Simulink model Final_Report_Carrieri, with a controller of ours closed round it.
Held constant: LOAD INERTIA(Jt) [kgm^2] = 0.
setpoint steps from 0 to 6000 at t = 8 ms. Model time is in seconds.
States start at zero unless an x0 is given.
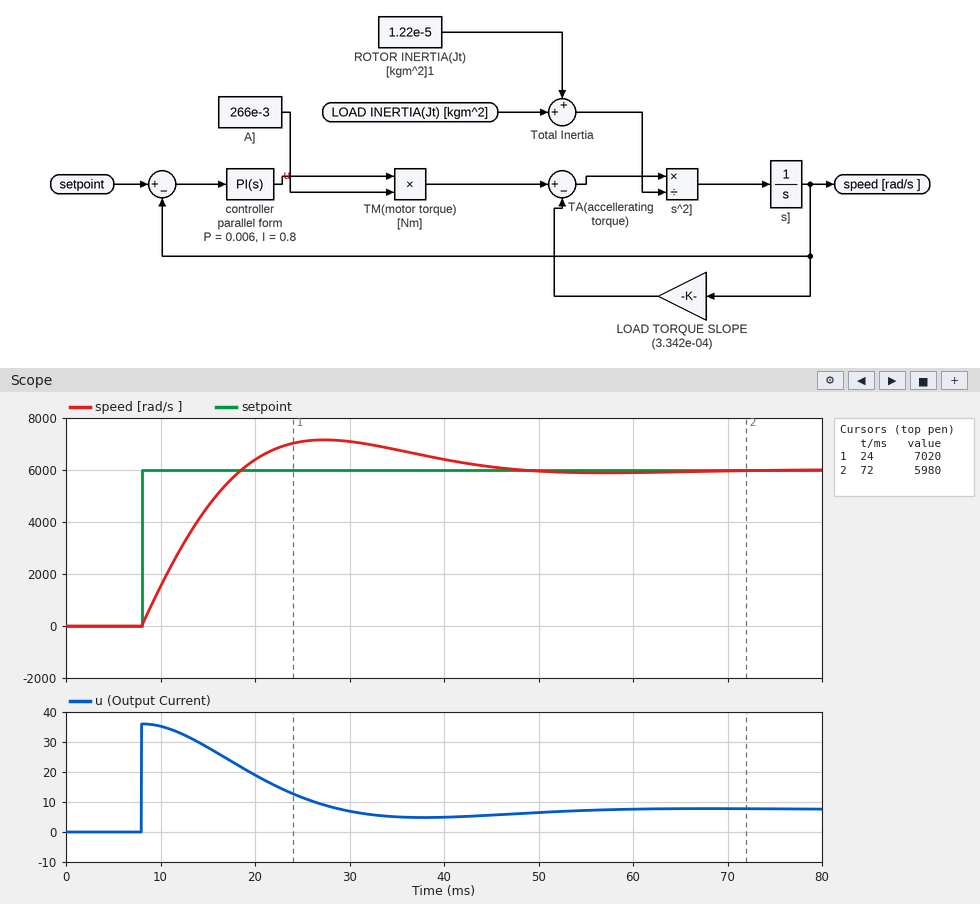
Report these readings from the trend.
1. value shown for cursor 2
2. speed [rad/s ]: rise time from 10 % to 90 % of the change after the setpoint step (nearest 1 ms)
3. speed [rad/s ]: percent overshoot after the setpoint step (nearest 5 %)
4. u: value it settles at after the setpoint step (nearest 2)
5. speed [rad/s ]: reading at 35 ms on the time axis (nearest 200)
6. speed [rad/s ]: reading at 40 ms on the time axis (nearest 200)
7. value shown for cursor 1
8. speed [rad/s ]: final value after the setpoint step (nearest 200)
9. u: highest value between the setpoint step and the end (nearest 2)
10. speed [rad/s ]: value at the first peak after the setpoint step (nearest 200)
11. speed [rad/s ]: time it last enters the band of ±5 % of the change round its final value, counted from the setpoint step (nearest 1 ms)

5980
8 ms
20 %
8
6800
6400
7020
6000
36
7200
34 ms
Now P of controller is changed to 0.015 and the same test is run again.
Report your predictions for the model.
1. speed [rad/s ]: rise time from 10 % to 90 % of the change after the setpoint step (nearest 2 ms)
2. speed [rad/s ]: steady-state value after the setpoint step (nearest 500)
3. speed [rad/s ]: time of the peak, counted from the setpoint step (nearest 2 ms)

6 ms
6000
16 ms
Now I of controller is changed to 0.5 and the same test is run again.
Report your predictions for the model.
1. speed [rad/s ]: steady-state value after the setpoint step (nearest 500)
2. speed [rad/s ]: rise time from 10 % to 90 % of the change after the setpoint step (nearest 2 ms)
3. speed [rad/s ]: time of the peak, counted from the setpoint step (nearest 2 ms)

6000
10 ms
24 ms
